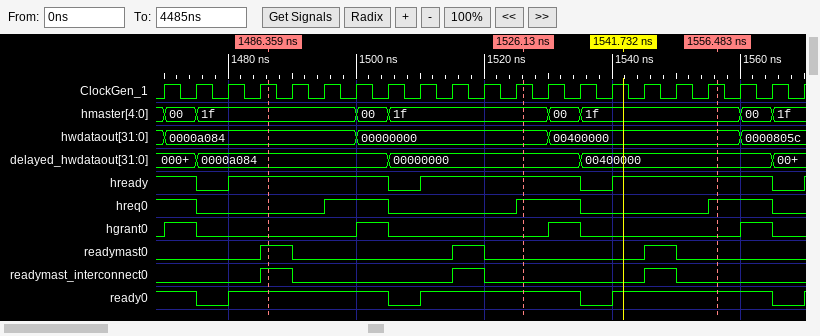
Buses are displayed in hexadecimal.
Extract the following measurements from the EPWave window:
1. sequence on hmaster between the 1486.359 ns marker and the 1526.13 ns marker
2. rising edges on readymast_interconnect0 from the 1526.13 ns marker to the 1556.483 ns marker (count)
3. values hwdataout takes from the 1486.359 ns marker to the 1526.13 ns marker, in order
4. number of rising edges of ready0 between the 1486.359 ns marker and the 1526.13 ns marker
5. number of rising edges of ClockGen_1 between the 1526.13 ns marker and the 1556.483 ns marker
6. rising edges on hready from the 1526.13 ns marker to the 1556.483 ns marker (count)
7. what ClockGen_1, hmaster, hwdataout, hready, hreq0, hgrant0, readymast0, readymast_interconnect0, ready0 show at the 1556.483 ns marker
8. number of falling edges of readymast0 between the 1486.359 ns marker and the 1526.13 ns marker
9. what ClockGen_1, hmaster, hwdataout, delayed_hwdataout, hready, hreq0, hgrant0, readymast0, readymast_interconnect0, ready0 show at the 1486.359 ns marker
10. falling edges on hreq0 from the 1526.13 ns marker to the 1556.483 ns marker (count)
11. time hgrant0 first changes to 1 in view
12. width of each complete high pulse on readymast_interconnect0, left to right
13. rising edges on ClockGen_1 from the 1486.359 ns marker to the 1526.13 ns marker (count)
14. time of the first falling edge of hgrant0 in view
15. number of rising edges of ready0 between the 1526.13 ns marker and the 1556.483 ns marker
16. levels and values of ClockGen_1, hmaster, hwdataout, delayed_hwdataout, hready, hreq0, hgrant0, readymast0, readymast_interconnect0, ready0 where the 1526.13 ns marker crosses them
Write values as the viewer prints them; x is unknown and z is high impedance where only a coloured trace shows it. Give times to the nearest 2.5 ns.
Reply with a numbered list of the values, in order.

1. 1f, 00, 1f
2. 1
3. 0000a084, 00000000
4. 1
5. 6
6. 1
7. ClockGen_1=1, hmaster=1f, hwdataout=00400000, hready=1, hreq0=1, hgrant0=0, readymast0=0, readymast_interconnect0=0, ready0=1
8. 2
9. ClockGen_1=1, hmaster=1f, hwdataout=0000a084, delayed_hwdataout=0000a084, hready=1, hreq0=0, hgrant0=0, readymast0=1, readymast_interconnect0=1, ready0=1
10. 1
11. 1470 ns
12. 5 ns, 5 ns, 5 ns
13. 8
14. 1475 ns
15. 1
16. ClockGen_1=1, hmaster=1f, hwdataout=00000000, delayed_hwdataout=00000000, hready=1, hreq0=1, hgrant0=0, readymast0=0, readymast_interconnect0=0, ready0=1
